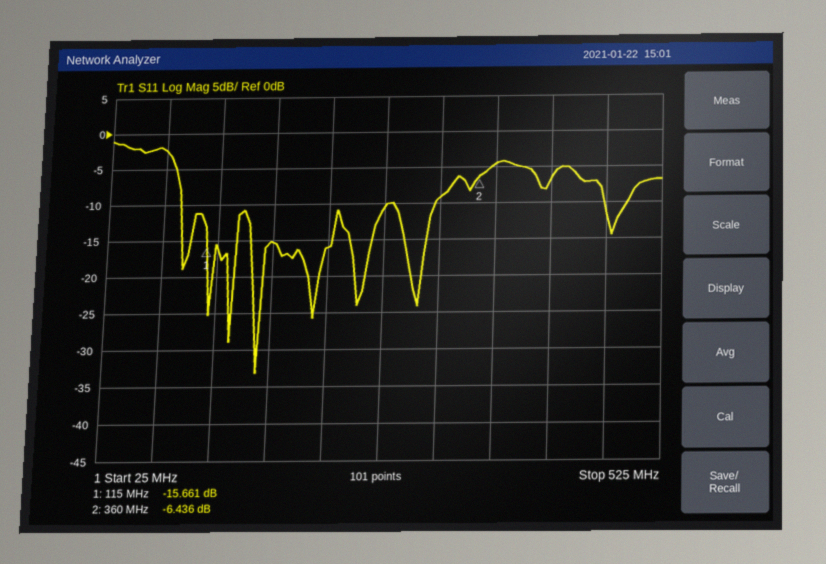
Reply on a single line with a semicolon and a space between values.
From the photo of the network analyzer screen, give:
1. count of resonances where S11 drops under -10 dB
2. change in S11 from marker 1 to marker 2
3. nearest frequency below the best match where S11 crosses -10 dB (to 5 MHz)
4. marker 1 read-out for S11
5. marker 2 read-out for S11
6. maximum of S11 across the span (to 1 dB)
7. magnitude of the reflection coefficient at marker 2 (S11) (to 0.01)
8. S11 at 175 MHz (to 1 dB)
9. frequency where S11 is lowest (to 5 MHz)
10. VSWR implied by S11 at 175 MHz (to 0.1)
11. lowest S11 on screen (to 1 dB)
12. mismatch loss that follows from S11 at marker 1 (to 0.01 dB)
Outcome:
8; 9.225 dB; 90 MHz; -15.661 dB; -6.436 dB; -1 dB; 0.48; -15 dB; 165 MHz; 1.4; -33 dB; 0.12 dB
